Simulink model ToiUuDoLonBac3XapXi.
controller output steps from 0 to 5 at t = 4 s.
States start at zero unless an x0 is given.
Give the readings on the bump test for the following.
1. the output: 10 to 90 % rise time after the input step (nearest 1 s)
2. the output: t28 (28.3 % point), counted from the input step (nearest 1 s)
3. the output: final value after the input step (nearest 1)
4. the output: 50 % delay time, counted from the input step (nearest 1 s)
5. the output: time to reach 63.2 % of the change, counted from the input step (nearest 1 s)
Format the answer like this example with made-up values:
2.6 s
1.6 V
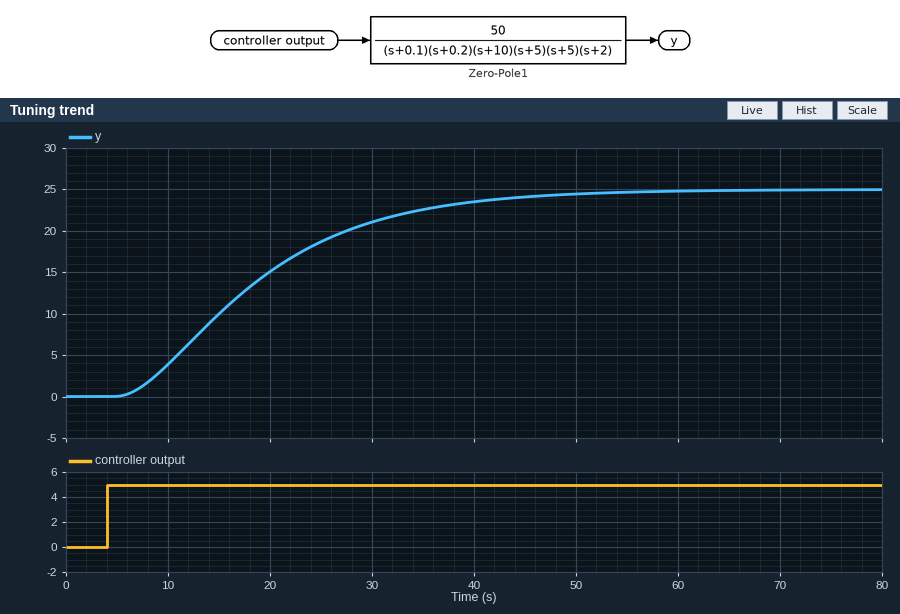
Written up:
26 s
9 s
25
13 s
17 s
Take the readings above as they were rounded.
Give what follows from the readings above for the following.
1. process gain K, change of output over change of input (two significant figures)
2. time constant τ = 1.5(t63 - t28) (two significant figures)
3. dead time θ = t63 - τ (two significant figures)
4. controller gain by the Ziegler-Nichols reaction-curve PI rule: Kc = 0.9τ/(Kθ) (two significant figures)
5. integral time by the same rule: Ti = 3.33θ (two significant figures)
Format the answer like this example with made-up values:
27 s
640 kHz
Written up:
5.0
12 s
5.0 s
0.43
17 s
